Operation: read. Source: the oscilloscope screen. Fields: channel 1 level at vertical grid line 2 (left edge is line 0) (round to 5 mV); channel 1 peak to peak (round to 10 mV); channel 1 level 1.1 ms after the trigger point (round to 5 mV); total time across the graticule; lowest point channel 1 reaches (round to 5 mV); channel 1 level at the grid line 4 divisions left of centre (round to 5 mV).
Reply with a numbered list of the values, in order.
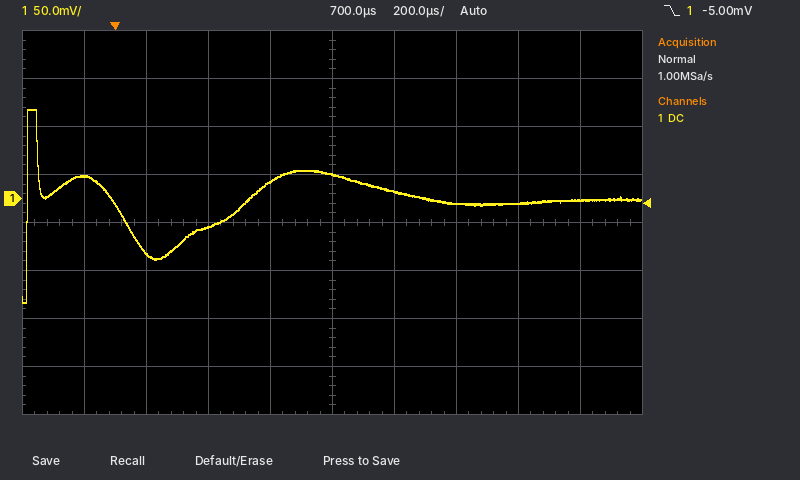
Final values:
1. -55 mV
2. 200 mV
3. -5 mV
4. 2 ms
5. -110 mV
6. 25 mV
